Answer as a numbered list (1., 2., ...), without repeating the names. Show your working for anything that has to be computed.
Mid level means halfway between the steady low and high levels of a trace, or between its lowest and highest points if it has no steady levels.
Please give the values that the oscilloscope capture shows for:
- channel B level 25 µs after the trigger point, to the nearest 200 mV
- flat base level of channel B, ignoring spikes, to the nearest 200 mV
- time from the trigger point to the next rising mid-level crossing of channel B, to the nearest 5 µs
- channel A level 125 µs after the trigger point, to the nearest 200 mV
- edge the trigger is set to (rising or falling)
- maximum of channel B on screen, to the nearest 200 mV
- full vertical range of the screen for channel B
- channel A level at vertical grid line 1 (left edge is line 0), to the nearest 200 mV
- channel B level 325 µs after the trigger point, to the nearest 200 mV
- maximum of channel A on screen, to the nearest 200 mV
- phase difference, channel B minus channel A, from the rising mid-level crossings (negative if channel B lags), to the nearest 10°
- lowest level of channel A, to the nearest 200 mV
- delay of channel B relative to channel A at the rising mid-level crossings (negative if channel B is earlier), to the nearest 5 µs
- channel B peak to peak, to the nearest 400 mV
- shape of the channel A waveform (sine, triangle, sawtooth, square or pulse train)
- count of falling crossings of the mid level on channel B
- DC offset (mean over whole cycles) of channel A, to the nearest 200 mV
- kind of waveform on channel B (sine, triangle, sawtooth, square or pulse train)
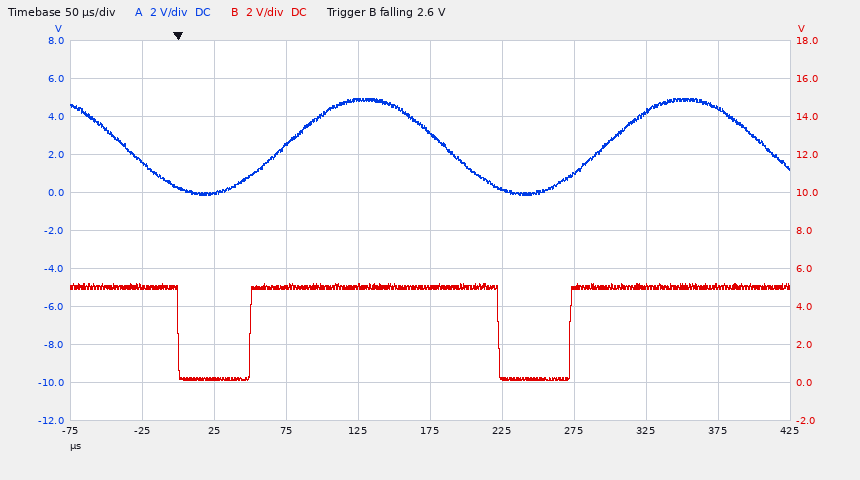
1. 200 mV
2. 200 mV
3. 50 µs
4. 4.8 V
5. falling
6. 5.2 V
7. 20 V
8. 1.6 V
9. 5.0 V
10. 5.0 V
11. +40°
12. -200 mV
13. -25 µs
14. 5.2 V
15. sine
16. 2
17. (5.0 V + (-200 mV)) / 2 ≈ 2.4 V
18. pulse train
